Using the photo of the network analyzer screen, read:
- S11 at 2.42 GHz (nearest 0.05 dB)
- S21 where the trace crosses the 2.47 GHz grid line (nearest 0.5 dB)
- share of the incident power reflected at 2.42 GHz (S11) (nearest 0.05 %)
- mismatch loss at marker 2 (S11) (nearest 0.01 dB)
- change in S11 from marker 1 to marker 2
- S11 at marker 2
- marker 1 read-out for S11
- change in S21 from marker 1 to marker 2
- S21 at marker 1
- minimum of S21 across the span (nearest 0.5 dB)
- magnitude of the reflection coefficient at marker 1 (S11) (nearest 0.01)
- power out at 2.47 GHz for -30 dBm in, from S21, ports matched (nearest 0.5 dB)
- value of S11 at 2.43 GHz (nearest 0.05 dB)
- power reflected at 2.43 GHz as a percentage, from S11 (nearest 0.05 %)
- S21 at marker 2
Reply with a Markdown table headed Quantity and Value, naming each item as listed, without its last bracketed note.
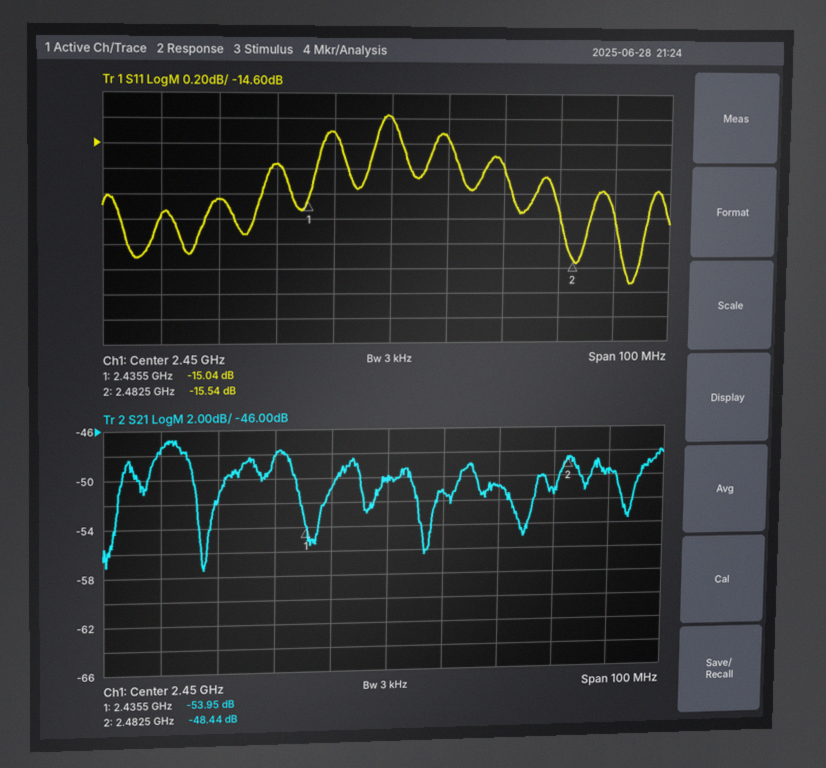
| Quantity | Value |
|---|---|
| S11 at 2.42 GHz | -15.05 dB |
| S21 where the trace crosses the 2.47 GHz grid line | -51.0 dB |
| share of the incident power reflected at 2.42 GHz (S11) | 3.15 % |
| mismatch loss at marker 2 (S11) | 0.12 dB |
| change in S11 from marker 1 to marker 2 | -0.50 dB |
| S11 at marker 2 | -15.54 dB |
| marker 1 read-out for S11 | -15.04 dB |
| change in S21 from marker 1 to marker 2 | 5.51 dB |
| S21 at marker 1 | -53.95 dB |
| minimum of S21 across the span | -57.5 dB |
| magnitude of the reflection coefficient at marker 1 (S11) | 0.18 |
| power out at 2.47 GHz for -30 dBm in, from S21, ports matched | -81.0 dBm |
| value of S11 at 2.43 GHz | -14.75 dB |
| power reflected at 2.43 GHz as a percentage, from S11 | 3.35 % |
| S21 at marker 2 | -48.44 dB |
